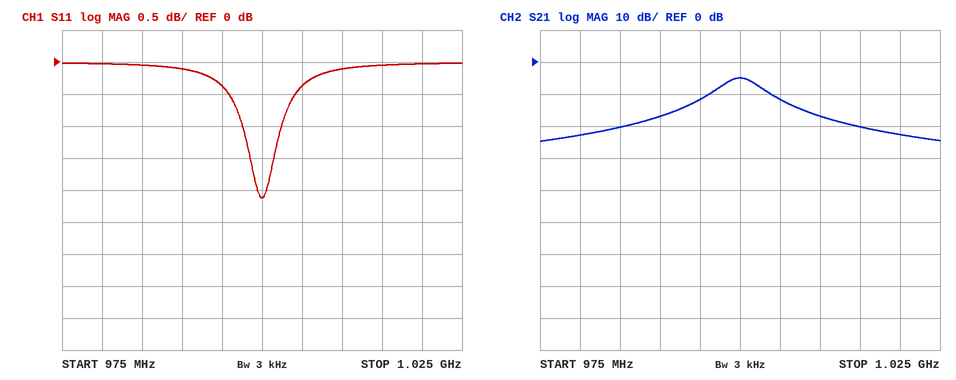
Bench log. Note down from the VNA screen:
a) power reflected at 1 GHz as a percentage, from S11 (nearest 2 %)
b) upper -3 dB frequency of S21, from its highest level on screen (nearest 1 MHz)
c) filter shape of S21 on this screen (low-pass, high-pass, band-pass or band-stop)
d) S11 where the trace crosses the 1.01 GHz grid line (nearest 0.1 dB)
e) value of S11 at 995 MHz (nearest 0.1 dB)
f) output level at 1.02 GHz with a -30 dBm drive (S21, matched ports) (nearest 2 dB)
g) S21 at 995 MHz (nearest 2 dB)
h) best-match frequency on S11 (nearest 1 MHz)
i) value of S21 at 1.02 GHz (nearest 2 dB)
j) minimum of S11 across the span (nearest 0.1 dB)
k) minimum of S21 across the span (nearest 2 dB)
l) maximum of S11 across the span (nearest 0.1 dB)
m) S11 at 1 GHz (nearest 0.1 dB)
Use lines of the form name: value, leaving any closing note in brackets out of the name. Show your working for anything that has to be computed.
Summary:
power reflected at 1 GHz as a percentage, from S11: 10^(-2.1/10) ≈ 62 %
upper -3 dB frequency of S21, from its highest level on screen: 1.003 GHz
filter shape of S21 on this screen: band-pass
S11 where the trace crosses the 1.01 GHz grid line: -0.1 dB
value of S11 at 995 MHz: -0.4 dB
output level at 1.02 GHz with a -30 dBm drive (S21, matched ports): -30 dBm + (-22 dB) = -52 dBm
S21 at 995 MHz: -12 dB
best-match frequency on S11: 1.000 GHz
value of S21 at 1.02 GHz: -22 dB
minimum of S11 across the span: -2.1 dB
minimum of S21 across the span: -24 dB
maximum of S11 across the span: 0.0 dB
S11 at 1 GHz: -2.1 dB
